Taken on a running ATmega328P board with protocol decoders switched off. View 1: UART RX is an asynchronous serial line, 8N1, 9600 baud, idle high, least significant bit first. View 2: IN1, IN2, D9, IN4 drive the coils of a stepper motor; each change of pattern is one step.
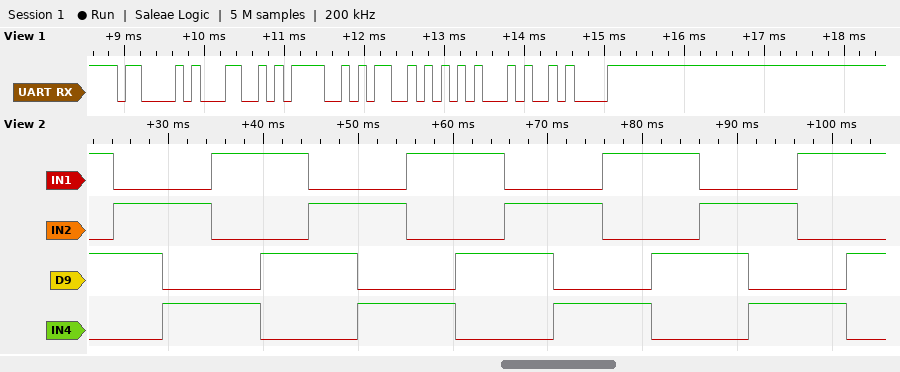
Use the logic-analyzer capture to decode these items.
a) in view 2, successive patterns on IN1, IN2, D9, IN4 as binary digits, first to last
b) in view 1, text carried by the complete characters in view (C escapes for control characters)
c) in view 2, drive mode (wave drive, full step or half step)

1010 0110 0101 1001 1010 0110 0101 1001 1010 0110 0101 1001 1010 0110 0101 1001 1010
"CLOSE\n"
full step
